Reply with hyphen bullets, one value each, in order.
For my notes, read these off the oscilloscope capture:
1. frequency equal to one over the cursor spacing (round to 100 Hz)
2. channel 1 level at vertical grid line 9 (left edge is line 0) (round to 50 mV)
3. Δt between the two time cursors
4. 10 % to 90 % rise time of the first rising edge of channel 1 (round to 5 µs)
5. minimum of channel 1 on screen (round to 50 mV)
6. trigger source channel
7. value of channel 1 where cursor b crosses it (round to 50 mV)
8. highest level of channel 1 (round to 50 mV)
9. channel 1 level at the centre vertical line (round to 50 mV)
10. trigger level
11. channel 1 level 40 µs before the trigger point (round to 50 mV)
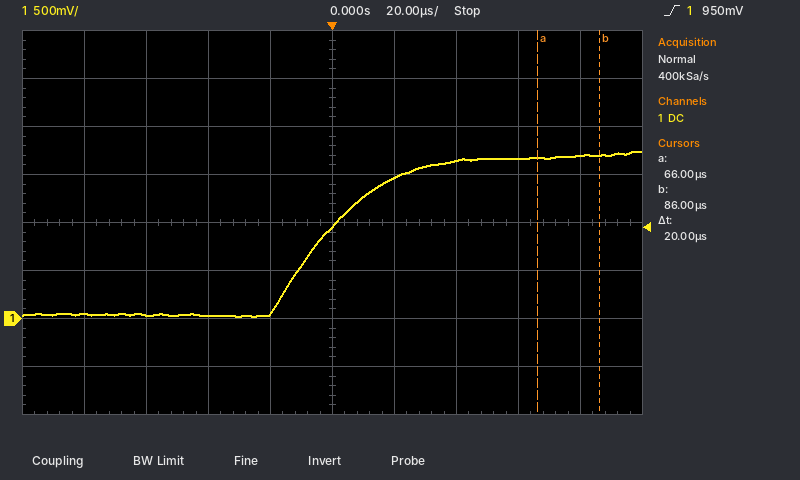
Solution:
- 50.0 kHz
- 1.70 V
- 20 µs
- 40 µs
- 0 mV
- channel 1
- 1.70 V
- 1.75 V
- 950 mV
- 950 mV
- 50 mV
